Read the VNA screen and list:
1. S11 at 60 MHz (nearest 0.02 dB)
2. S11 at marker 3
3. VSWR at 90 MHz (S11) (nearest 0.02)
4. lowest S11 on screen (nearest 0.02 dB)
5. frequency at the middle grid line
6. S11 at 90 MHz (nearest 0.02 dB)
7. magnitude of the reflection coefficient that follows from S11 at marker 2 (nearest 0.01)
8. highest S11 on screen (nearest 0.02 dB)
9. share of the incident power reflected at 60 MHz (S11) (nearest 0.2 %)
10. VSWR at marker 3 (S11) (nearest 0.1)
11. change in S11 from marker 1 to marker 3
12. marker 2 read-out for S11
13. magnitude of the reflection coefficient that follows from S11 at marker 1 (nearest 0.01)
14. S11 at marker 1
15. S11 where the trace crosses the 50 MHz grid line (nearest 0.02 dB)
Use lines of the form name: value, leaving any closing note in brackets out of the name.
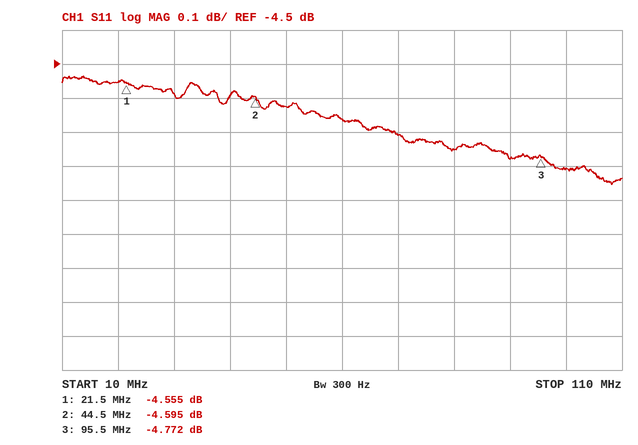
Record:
S11 at 60 MHz: -4.66 dB
S11 at marker 3: -4.772 dB
VSWR at 90 MHz (S11): 3.72
lowest S11 on screen: -4.86 dB
frequency at the middle grid line: 60 MHz
S11 at 90 MHz: -4.78 dB
magnitude of the reflection coefficient that follows from S11 at marker 2: 0.59
highest S11 on screen: -4.54 dB
share of the incident power reflected at 60 MHz (S11): 34.2 %
VSWR at marker 3 (S11): 3.7
change in S11 from marker 1 to marker 3: -0.217 dB
marker 2 read-out for S11: -4.595 dB
magnitude of the reflection coefficient that follows from S11 at marker 1: 0.59
S11 at marker 1: -4.555 dB
S11 where the trace crosses the 50 MHz grid line: -4.62 dB
